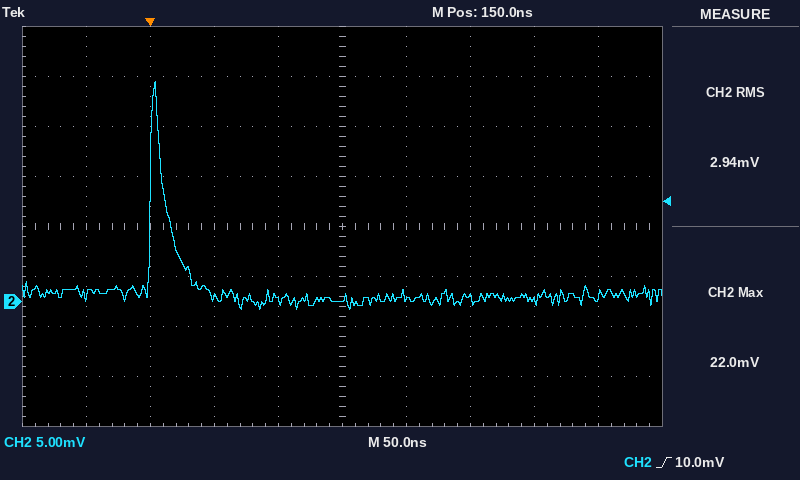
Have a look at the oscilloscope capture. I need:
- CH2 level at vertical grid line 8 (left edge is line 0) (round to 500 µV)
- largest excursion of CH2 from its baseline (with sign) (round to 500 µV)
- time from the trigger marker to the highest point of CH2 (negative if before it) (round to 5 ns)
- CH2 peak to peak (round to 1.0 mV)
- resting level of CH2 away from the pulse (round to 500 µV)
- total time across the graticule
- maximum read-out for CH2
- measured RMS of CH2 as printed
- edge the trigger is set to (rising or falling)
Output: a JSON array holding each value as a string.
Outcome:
["0.0 mV", "+21.5 mV", "+5 ns", "23.0 mV", "500 µV", "500 ns", "22.0 mV", "2.94 mV", "rising"]
